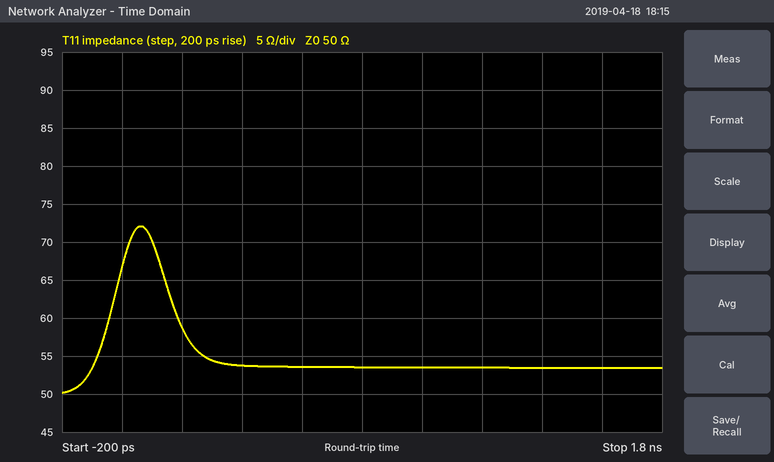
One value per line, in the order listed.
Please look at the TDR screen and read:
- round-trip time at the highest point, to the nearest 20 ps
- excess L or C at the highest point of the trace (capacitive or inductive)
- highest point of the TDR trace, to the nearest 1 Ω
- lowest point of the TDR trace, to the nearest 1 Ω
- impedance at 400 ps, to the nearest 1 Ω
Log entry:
60 ps
inductive
72 Ω
50 Ω
54 Ω
